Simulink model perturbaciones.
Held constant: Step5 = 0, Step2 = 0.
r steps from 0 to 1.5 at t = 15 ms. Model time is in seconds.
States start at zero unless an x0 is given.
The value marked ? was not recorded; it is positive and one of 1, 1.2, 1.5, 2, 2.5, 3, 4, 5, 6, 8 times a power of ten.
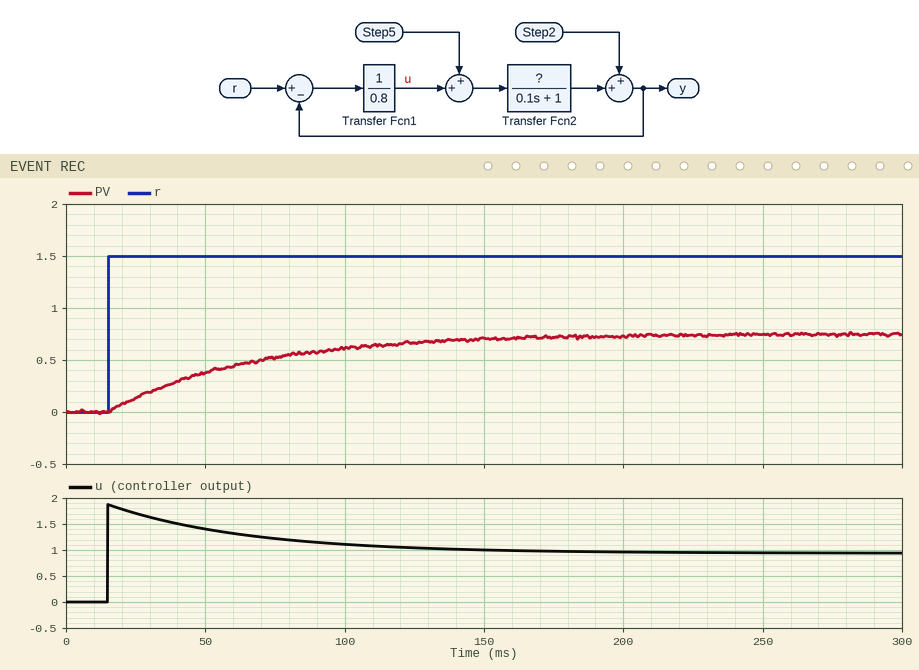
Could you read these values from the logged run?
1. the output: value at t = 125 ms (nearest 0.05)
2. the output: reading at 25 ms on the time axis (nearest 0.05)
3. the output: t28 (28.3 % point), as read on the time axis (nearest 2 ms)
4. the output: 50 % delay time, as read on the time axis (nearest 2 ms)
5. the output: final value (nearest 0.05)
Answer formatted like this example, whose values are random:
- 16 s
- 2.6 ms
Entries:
- 0.65
- 0.15
- 32 ms
- 50 ms
- 0.75
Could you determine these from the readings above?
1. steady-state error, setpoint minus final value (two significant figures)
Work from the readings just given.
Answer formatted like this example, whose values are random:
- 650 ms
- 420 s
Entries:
- 0.75
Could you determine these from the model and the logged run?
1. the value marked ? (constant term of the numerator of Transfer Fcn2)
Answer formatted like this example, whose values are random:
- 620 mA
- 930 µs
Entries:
- 0.8
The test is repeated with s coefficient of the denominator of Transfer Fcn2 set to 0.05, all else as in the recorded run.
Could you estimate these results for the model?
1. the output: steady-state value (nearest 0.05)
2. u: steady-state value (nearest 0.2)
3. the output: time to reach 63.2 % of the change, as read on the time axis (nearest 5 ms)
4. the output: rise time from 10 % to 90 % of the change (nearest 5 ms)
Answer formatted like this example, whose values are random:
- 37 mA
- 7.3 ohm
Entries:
- 0.75
- 1.0
- 40 ms
- 55 ms
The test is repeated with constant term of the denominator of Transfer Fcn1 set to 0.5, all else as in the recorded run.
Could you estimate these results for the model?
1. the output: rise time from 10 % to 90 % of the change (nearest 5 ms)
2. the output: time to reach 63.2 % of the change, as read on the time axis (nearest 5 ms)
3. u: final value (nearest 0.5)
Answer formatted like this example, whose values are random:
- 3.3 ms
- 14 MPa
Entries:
- 85 ms
- 55 ms
- 1.0
